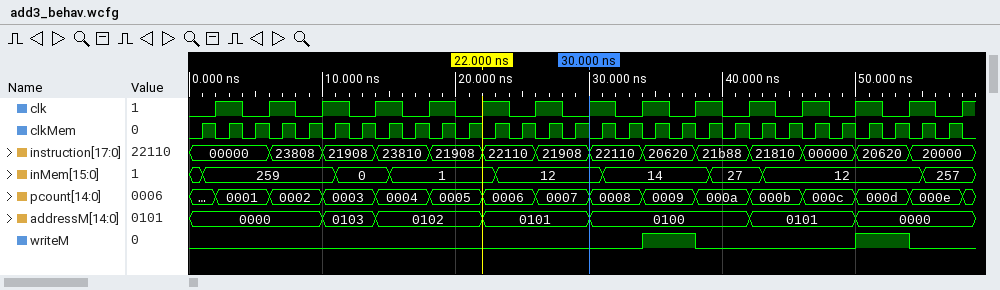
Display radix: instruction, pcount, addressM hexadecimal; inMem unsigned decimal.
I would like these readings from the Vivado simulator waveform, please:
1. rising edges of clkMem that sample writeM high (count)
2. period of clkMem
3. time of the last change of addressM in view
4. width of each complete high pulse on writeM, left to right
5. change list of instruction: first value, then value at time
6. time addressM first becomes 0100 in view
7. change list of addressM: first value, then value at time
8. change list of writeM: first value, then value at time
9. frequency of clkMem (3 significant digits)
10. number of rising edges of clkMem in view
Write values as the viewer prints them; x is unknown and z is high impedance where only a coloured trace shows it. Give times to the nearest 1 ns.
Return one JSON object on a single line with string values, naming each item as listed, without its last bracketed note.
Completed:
{"rising edges of clkMem that sample writeM high": "4", "period of clkMem": "2 ns", "time of the last change of addressM in view": "50 ns", "width of each complete high pulse on writeM, left to right": "4 ns, 4 ns", "change list of instruction: first value, then value at time": "00000, 23808 at 6 ns, 21908 at 10 ns, 23810 at 14 ns, 21908 at 18 ns, 22110 at 22 ns, 21908 at 26 ns, 22110 at 30 ns, 20620 at 34 ns, 21b88 at 38 ns, 21810 at 42 ns, 00000 at 46 ns, 20620 at 50 ns, 20000 at 54 ns", "time addressM first becomes 0100 in view": "30 ns", "change list of addressM: first value, then value at time": "0000, 0103 at 10 ns, 0102 at 14 ns, 0101 at 22 ns, 0100 at 30 ns, 0101 at 42 ns, 0000 at 50 ns", "change list of writeM: first value, then value at time": "0, 1 at 34 ns, 0 at 38 ns, 1 at 50 ns, 0 at 54 ns", "frequency of clkMem": "500 MHz", "number of rising edges of clkMem in view": "29"}
